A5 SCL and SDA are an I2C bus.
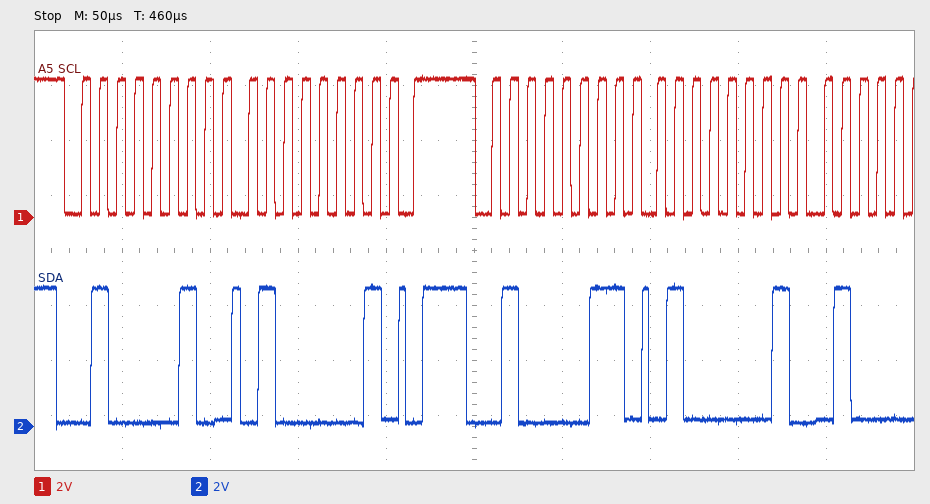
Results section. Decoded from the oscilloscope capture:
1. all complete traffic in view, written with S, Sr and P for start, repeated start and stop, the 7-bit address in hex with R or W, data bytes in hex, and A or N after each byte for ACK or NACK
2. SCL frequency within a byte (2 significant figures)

S 21W A 41 A P S 21R A 41 A
100 kHz
